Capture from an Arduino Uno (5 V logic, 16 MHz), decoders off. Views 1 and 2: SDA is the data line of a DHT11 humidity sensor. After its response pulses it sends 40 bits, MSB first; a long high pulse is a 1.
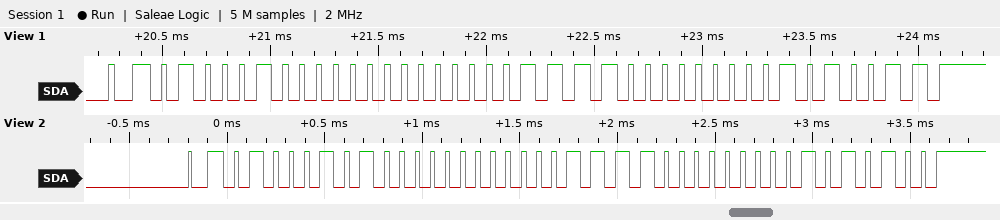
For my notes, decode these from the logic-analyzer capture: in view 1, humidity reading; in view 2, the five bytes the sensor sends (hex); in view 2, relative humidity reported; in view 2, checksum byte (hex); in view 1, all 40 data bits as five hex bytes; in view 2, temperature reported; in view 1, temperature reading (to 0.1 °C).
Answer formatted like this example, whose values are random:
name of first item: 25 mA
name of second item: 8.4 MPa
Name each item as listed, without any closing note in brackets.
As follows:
in view 1, humidity reading: 68 %
in view 2, the five bytes the sensor sends: 45 00 0F 00 54
in view 2, relative humidity reported: 69 %
in view 2, checksum byte: 0x54
in view 1, all 40 data bits as five hex bytes: 44 00 0F 00 53
in view 2, temperature reported: 15.0 °C
in view 1, temperature reading: 15.0 °C
